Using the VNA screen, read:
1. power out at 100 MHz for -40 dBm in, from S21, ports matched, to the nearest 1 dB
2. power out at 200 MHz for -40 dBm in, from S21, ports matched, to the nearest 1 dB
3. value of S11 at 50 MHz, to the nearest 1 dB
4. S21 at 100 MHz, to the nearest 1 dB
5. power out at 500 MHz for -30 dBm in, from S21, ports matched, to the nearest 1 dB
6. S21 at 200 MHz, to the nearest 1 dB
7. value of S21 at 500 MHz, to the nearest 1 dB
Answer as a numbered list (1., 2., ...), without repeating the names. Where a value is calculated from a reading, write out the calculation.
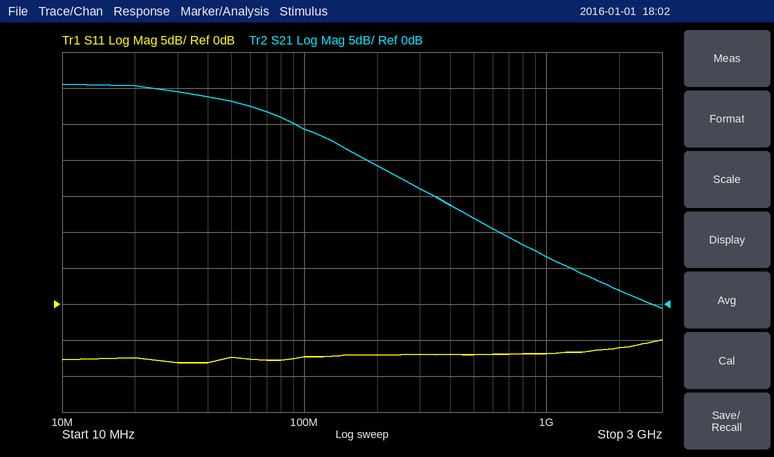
1. -40 dBm + (24 dB) = -16 dBm
2. -40 dBm + (19 dB) = -21 dBm
3. -7 dB
4. 24 dB
5. -30 dBm + (12 dB) = -18 dBm
6. 19 dB
7. 12 dB
